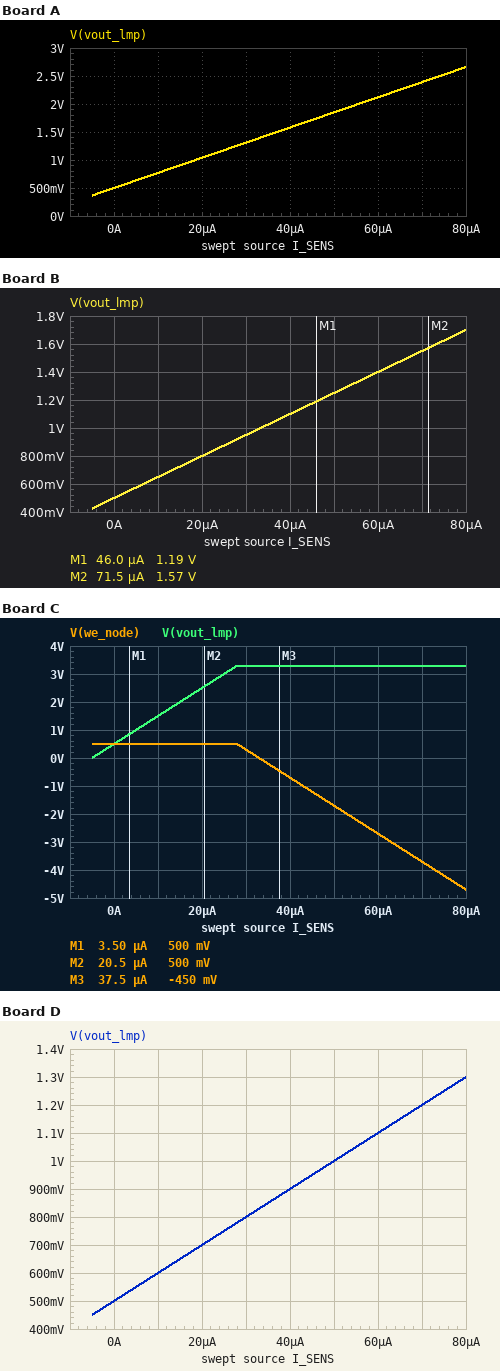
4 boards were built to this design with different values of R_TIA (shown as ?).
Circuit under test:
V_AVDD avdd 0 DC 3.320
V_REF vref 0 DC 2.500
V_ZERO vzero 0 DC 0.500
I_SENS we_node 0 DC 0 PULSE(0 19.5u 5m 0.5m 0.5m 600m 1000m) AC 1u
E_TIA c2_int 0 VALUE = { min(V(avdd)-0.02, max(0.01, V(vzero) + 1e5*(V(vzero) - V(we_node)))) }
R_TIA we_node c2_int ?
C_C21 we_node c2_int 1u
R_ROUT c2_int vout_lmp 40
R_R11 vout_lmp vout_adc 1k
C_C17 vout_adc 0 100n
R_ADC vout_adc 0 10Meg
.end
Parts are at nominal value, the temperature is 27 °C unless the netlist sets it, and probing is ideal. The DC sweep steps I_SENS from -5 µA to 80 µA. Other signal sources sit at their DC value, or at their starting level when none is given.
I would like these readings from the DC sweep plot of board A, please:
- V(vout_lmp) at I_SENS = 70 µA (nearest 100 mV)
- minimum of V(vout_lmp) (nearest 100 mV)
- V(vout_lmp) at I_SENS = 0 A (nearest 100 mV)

2.4 V
400 mV
500 mV
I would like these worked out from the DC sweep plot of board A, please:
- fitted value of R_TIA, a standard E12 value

27 kΩ
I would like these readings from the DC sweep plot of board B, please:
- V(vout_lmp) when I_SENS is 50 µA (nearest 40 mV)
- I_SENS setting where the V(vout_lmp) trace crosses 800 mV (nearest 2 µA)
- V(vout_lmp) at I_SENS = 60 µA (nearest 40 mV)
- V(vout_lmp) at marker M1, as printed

1.24 V
20 µA
1.40 V
1.19 V
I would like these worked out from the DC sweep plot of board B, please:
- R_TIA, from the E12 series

15 kΩ
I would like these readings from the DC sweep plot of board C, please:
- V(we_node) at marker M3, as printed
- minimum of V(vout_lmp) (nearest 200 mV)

-450 mV
0 V
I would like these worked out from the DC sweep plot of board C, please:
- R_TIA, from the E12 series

100 kΩ
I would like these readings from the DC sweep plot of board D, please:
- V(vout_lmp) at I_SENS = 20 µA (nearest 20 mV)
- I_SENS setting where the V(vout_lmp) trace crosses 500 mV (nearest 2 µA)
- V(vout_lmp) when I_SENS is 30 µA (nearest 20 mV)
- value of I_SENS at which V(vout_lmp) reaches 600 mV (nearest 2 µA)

700 mV
0 A
800 mV
10 µA
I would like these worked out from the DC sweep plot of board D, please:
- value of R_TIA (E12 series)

10 kΩ
